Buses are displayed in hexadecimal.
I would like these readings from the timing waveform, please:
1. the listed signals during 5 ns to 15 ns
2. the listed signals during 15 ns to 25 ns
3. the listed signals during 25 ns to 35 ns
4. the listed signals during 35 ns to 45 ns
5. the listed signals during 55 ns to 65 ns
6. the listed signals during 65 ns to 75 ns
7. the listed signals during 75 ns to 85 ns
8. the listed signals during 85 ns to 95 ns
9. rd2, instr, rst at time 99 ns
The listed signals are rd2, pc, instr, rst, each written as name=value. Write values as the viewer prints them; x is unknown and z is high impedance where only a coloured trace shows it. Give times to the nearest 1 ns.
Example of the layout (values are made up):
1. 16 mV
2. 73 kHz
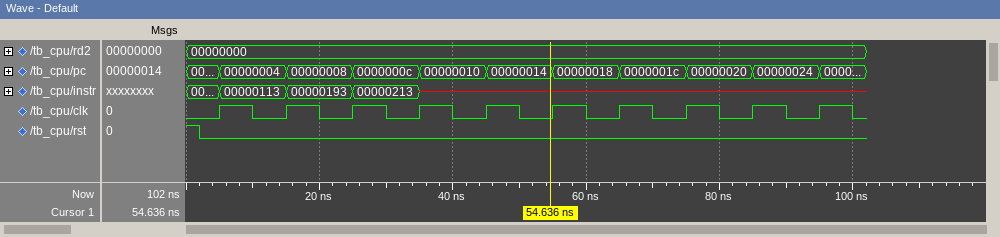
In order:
1. rd2=00000000, pc=00000004, instr=00000113, rst=0
2. rd2=00000000, pc=00000008, instr=00000193, rst=0
3. rd2=00000000, pc=0000000c, instr=00000213, rst=0
4. rd2=00000000, pc=00000010, instr=x, rst=0
5. rd2=00000000, pc=00000018, instr=x, rst=0
6. rd2=00000000, pc=0000001c, instr=x, rst=0
7. rd2=00000000, pc=00000020, instr=x, rst=0
8. rd2=00000000, pc=00000024, instr=x, rst=0
9. rd2=00000000, instr=x, rst=0
